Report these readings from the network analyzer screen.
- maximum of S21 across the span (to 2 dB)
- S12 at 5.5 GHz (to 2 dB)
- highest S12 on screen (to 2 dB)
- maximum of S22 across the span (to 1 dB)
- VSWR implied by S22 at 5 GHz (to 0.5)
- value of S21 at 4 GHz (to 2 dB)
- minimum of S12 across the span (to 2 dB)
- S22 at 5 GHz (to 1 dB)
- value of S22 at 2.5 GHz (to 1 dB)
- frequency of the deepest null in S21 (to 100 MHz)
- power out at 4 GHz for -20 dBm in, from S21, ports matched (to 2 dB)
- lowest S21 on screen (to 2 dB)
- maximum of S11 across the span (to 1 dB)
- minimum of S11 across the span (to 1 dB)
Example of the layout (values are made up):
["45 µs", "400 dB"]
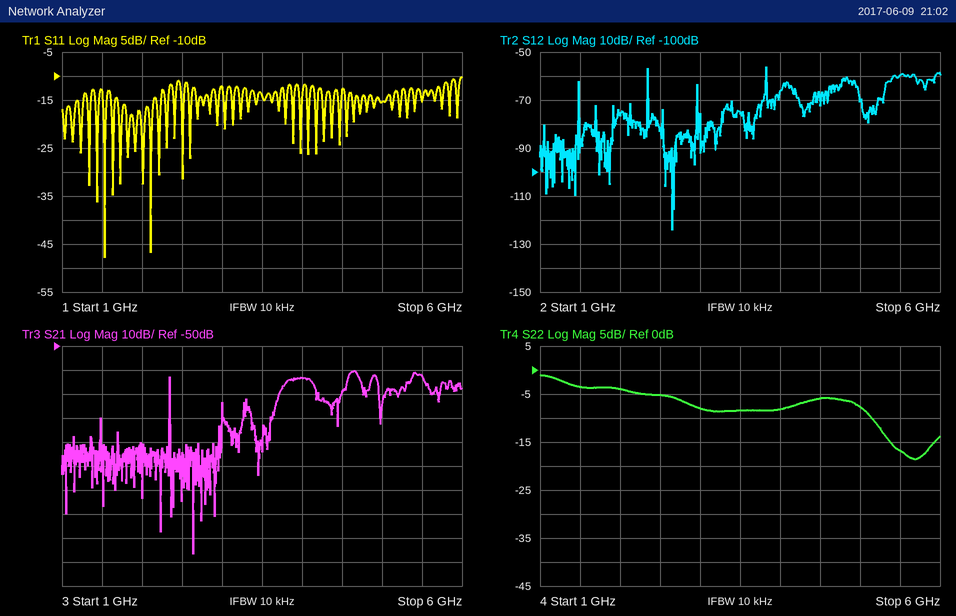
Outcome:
["-60 dB", "-60 dB", "-56 dB", "-1 dB", "2.5", "-64 dB", "-124 dB", "-8 dB", "-5 dB", "2.6 GHz", "-84 dBm", "-136 dB", "-10 dB", "-48 dB"]
